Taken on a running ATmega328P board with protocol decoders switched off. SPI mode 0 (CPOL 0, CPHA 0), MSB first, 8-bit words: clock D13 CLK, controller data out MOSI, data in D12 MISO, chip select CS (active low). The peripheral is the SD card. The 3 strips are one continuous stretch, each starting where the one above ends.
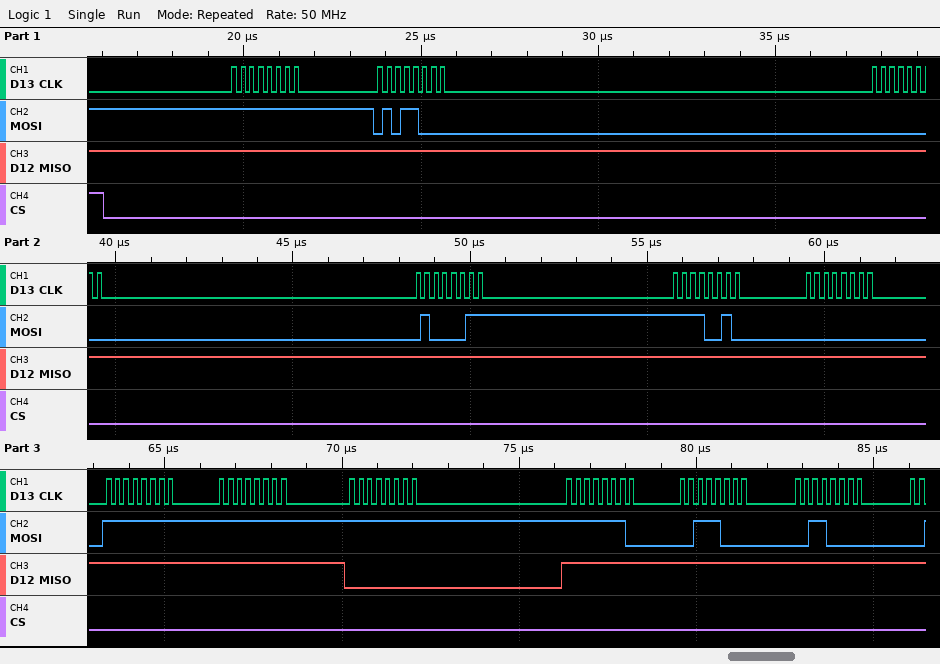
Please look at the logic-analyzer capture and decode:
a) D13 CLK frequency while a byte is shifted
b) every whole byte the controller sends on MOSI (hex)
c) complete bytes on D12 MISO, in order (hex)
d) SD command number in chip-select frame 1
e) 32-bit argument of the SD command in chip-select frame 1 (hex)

4 MHz
0xFF 0x58 0x00 0x43 0xF2 0x00 0xFF 0xFF 0xFF 0xFE 0x38 0x30
0xFF 0xFF 0xFF 0xFF 0xFF 0xFF 0xFF 0xFF 0x00 0xFF 0xFF 0xFF
CMD24
0x0043F200
